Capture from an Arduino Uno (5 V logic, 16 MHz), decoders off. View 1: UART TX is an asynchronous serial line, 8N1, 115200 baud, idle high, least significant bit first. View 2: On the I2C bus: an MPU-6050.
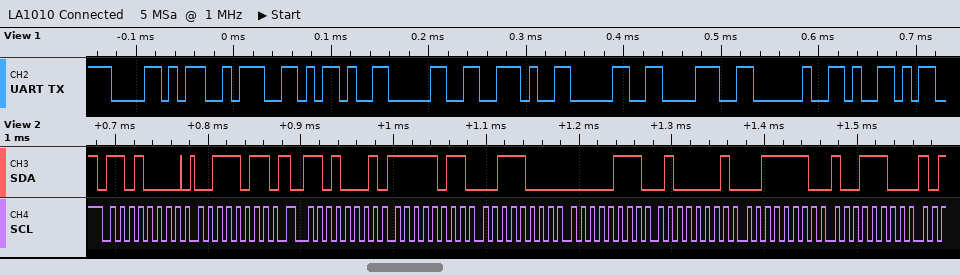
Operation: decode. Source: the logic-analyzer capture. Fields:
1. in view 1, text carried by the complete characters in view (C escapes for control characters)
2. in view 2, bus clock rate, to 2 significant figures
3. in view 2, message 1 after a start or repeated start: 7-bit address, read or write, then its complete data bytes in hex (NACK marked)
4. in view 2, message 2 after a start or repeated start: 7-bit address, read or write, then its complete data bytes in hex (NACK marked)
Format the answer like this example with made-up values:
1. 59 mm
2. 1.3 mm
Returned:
1. "X:-0.08 Y"
2. 100 kHz
3. 0x68 write: 3B
4. 0x68 read: FB 38 07 41 3E 9C
